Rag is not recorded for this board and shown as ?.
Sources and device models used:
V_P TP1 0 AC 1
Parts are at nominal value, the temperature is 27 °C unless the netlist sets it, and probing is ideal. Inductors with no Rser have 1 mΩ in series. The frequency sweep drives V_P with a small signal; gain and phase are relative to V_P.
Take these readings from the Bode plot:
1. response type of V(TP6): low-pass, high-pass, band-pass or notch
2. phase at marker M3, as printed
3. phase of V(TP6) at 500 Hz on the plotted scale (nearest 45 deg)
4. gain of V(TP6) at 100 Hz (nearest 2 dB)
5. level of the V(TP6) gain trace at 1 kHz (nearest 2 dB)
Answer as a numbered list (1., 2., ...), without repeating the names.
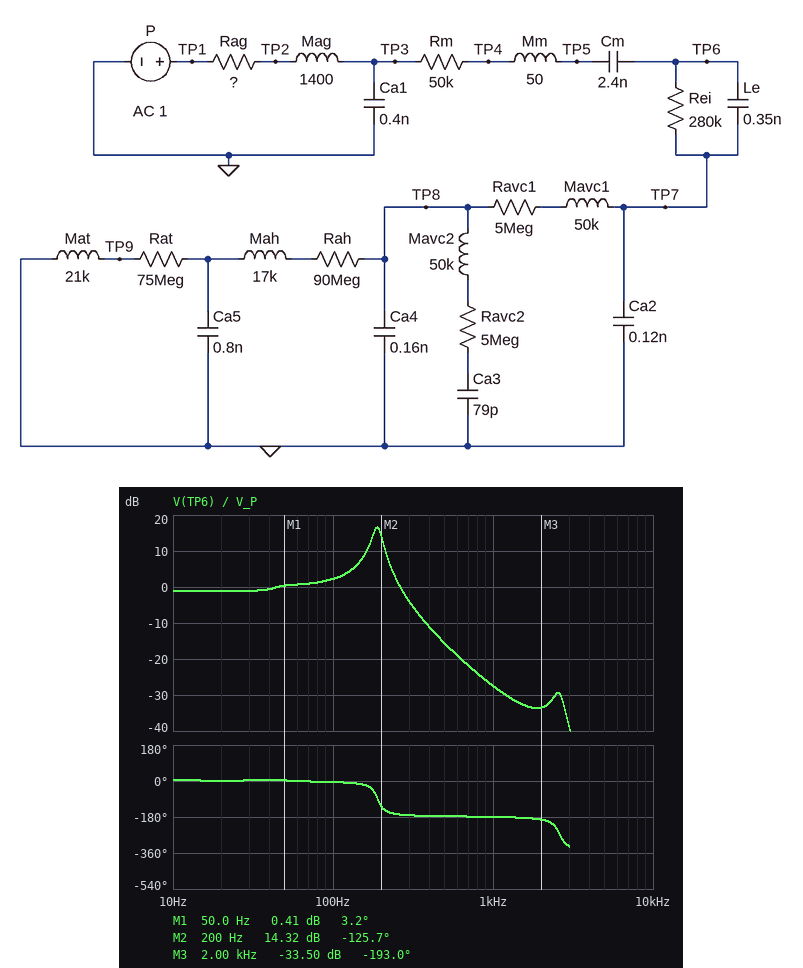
1. low-pass
2. -193.0 deg
3. -180 deg
4. 2 dB
5. -28 dB
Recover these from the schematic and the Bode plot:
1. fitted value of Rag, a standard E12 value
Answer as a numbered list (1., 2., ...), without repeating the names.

1. 220 kΩ
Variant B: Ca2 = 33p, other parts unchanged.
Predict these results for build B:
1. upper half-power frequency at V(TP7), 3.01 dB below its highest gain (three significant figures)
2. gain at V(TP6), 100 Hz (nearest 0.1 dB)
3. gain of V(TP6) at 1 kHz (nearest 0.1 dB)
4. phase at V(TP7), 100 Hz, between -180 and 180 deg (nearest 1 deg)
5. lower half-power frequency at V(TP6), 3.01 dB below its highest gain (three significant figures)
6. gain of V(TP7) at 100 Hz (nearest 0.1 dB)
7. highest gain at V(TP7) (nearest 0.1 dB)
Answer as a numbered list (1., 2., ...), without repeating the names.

1. 219 Hz
2. 2.1 dB
3. -26.8 dB
4. -5 deg
5. 194 Hz
6. 2.0 dB
7. 18.1 dB
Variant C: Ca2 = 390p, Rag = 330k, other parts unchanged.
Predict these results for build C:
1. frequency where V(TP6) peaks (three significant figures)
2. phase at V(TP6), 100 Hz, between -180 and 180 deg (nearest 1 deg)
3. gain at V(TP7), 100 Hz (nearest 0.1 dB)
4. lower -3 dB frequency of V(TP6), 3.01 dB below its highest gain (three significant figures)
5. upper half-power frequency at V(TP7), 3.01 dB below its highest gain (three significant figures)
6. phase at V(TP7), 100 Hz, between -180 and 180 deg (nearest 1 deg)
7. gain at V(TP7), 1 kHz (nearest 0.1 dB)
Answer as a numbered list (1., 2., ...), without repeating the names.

1. 156 Hz
2. -15 deg
3. 2.6 dB
4. 132 Hz
5. 176 Hz
6. -18 deg
7. -31.7 dB
